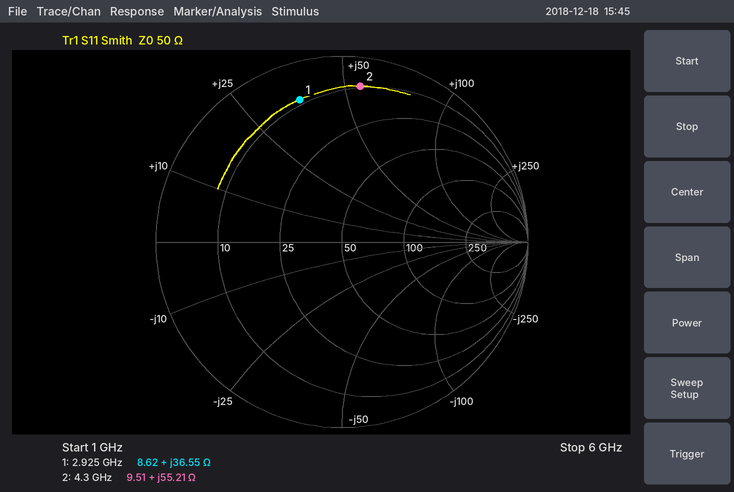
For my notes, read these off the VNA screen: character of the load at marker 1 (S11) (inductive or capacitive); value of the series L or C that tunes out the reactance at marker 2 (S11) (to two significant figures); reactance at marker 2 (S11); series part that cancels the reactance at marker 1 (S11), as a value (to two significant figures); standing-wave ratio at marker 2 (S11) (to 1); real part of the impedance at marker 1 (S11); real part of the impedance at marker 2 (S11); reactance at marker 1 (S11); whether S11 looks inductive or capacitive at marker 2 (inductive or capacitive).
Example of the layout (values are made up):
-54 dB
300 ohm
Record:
inductive
670 fF
+55.21 Ω
1.5 pF
12
8.62 Ω
9.51 Ω
+36.55 Ω
inductive
